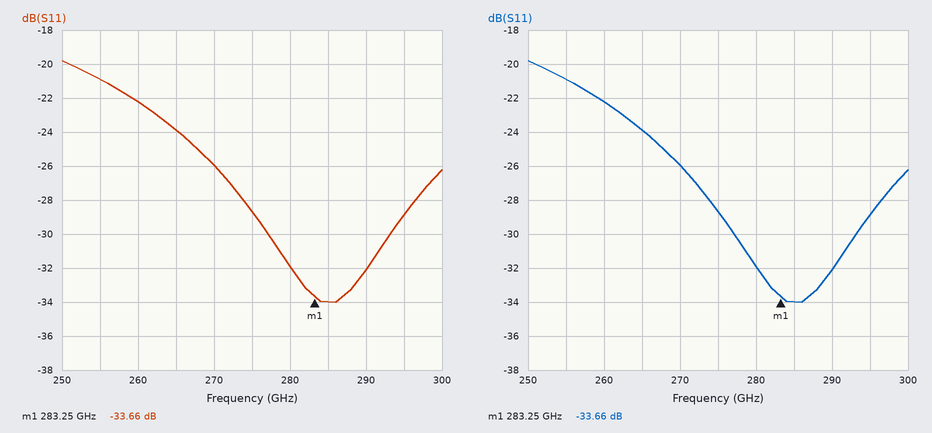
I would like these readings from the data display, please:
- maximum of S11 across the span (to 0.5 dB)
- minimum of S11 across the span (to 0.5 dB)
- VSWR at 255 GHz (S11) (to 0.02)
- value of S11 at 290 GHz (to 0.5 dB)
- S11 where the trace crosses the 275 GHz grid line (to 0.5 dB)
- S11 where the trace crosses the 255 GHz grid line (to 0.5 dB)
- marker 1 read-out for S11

-20.0 dB
-34.0 dB
1.20
-32.0 dB
-28.5 dB
-21.0 dB
-33.66 dB
